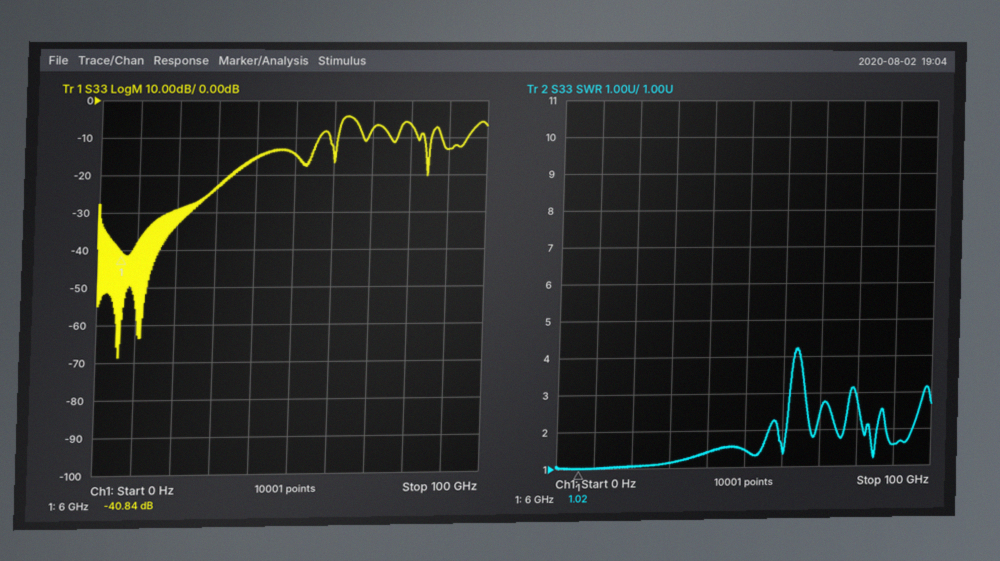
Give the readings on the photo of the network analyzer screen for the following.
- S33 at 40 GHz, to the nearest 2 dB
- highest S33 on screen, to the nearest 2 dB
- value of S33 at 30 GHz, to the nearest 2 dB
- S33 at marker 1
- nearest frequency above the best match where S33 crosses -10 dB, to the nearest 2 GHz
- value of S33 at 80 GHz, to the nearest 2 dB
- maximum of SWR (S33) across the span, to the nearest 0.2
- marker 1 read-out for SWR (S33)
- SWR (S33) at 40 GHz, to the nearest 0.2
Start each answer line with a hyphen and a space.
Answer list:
- -16 dB
- -4 dB
- -24 dB
- -40.84 dB
- 56 GHz
- -6 dB
- 4.2
- 1.02
- 1.4
